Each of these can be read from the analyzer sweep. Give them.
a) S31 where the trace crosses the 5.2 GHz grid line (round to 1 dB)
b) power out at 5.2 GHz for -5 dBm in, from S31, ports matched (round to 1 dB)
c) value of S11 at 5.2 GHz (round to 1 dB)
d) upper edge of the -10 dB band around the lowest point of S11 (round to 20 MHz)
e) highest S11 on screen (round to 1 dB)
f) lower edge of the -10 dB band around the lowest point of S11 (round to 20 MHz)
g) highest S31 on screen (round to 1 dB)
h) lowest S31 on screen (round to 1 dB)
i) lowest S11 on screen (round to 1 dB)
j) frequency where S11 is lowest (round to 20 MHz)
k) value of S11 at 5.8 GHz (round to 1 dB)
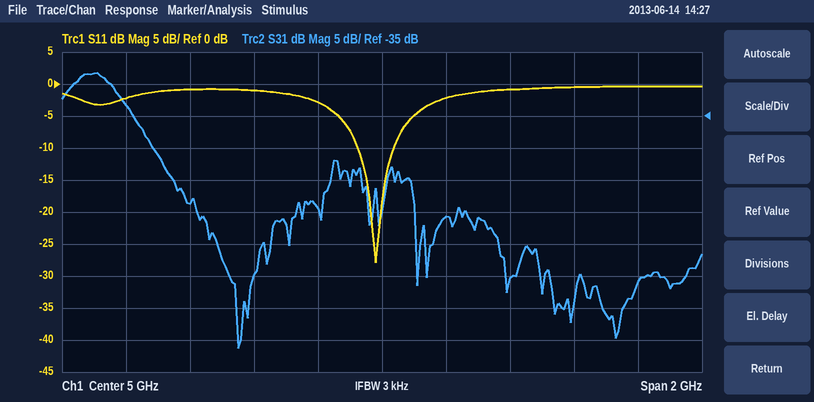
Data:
-51 dB
-56 dBm
-2 dB
5.04 GHz
0 dB
4.92 GHz
-28 dB
-71 dB
-28 dB
4.98 GHz
0 dB
